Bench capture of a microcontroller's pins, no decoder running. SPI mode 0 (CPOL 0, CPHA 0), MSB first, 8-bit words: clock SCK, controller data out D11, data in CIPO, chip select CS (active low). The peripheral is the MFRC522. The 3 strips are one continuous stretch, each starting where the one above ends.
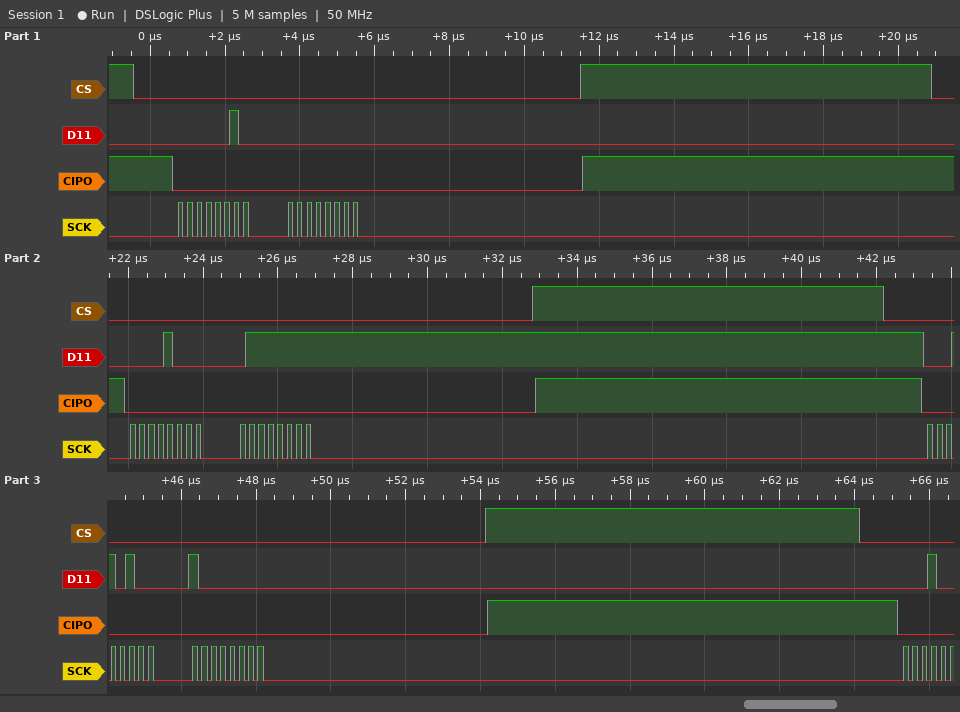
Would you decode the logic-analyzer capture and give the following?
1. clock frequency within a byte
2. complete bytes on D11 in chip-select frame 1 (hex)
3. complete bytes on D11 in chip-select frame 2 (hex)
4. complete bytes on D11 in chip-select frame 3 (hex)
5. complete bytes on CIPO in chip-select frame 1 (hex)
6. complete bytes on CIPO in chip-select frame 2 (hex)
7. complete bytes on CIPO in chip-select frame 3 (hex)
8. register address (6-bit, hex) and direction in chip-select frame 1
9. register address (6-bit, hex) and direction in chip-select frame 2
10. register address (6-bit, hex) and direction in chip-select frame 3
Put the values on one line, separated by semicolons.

4 MHz; 0x02 0x00; 0x08 0x7F; 0x14 0x80; 0x00 0x00; 0x00 0x00; 0x00 0x00; 0x01 write; 0x04 write; 0x0A write
